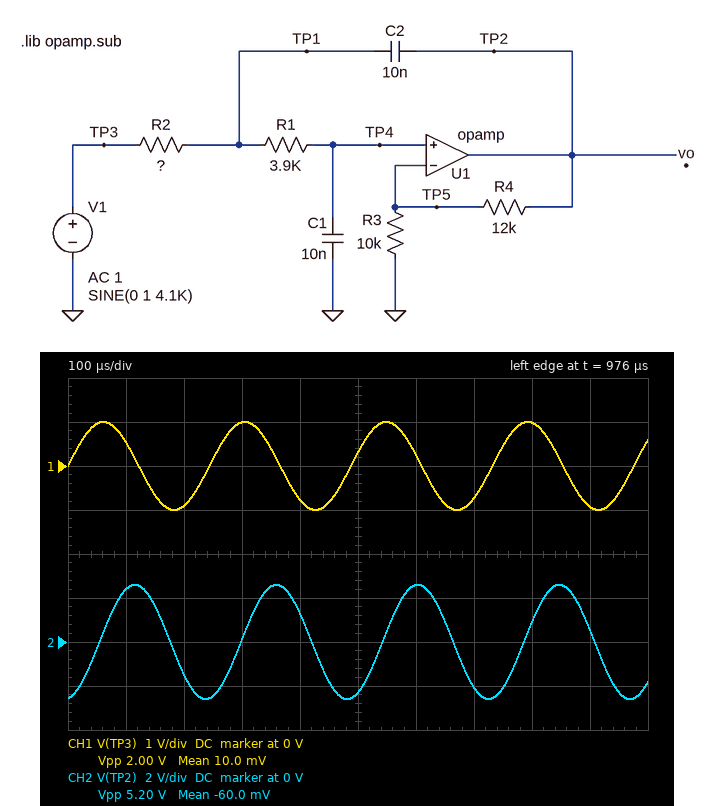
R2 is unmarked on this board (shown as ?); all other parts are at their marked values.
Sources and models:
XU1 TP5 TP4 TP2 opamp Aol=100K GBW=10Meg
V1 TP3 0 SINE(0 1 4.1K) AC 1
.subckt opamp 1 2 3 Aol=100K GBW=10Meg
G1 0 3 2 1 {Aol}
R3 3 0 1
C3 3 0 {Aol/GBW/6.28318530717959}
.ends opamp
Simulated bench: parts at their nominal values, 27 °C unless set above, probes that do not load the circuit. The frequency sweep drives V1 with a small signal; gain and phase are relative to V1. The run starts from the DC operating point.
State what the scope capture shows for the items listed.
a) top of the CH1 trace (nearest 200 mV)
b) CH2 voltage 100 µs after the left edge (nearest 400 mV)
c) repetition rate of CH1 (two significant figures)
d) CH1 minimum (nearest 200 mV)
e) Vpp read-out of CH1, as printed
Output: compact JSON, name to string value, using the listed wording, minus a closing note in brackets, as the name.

{"top of the CH1 trace": "1.0 V", "CH2 voltage 100 µs after the left edge": "2.4 V", "repetition rate of CH1": "4.1 kHz", "CH1 minimum": "-1.0 V", "Vpp read-out of CH1, as printed": "2.00 V"}
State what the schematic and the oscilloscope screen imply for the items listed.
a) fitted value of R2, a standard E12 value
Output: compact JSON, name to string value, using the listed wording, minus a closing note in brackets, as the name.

{"fitted value of R2, a standard E12 value": "3.3 kΩ"}
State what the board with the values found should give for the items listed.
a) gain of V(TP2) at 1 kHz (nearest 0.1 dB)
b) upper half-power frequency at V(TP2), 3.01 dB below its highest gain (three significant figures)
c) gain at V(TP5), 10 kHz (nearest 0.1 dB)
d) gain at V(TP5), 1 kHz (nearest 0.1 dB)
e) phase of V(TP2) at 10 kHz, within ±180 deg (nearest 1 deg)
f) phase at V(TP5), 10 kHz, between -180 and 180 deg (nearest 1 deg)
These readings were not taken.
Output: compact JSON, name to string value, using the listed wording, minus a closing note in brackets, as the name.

{"gain of V(TP2) at 1 kHz": "7.1 dB", "upper half-power frequency at V(TP2), 3.01 dB below its highest gain": "5.24 kHz", "gain at V(TP5), 10 kHz": "-13.2 dB", "gain at V(TP5), 1 kHz": "0.3 dB", "phase of V(TP2) at 10 kHz, within ±180 deg": "-154 deg", "phase at V(TP5), 10 kHz, between -180 and 180 deg": "-154 deg"}
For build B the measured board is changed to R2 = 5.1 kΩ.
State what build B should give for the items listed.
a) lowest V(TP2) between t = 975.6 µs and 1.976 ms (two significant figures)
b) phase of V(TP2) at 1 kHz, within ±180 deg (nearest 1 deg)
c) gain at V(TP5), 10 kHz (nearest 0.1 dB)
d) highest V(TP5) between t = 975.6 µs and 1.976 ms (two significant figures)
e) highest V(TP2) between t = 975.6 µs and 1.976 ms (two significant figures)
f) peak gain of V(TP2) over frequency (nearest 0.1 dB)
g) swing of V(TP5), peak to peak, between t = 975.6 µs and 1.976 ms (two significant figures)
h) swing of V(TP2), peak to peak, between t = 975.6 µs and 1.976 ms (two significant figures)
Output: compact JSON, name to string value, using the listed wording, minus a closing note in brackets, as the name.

{"lowest V(TP2) between t = 975.6 µs and 1.976 ms": "-2.7 V", "phase of V(TP2) at 1 kHz, within ±180 deg": "-11 deg", "gain at V(TP5), 10 kHz": "-17.0 dB", "highest V(TP5) between t = 975.6 µs and 1.976 ms": "1.2 V", "highest V(TP2) between t = 975.6 µs and 1.976 ms": "2.7 V", "peak gain of V(TP2) over frequency": "11.1 dB", "swing of V(TP5), peak to peak, between t = 975.6 µs and 1.976 ms": "2.5 V", "swing of V(TP2), peak to peak, between t = 975.6 µs and 1.976 ms": "5.4 V"}
